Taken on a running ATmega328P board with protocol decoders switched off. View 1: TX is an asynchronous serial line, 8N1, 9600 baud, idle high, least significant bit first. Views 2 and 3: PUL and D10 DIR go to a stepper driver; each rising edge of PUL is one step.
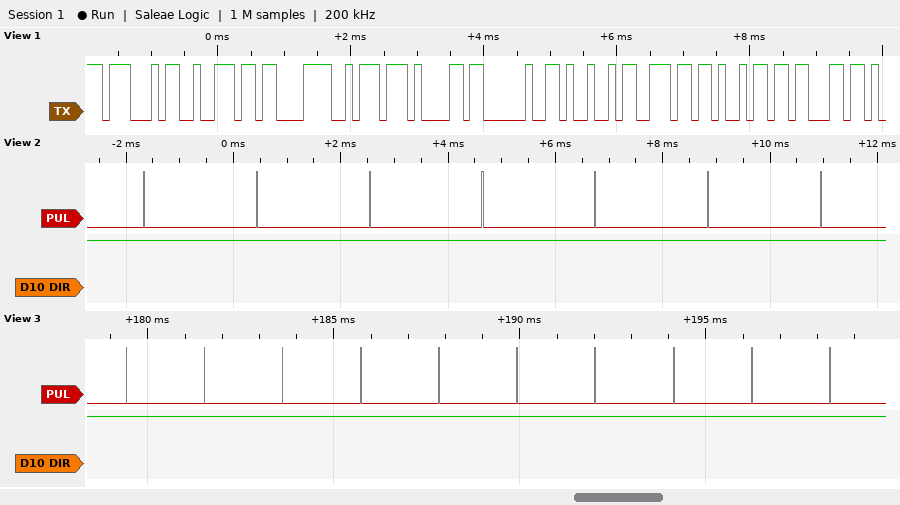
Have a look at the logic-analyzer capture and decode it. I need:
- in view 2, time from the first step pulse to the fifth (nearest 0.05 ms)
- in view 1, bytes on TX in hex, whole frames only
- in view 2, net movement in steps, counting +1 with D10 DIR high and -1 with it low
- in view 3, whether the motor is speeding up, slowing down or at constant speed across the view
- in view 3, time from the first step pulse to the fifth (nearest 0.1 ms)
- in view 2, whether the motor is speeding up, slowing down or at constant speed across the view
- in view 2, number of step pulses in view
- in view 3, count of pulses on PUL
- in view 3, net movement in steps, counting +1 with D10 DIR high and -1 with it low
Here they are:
8.40 ms
47 72 C3 BA 61 20 49 6E 69 63
+7
constant speed
8.4 ms
constant speed
7
10
+10
